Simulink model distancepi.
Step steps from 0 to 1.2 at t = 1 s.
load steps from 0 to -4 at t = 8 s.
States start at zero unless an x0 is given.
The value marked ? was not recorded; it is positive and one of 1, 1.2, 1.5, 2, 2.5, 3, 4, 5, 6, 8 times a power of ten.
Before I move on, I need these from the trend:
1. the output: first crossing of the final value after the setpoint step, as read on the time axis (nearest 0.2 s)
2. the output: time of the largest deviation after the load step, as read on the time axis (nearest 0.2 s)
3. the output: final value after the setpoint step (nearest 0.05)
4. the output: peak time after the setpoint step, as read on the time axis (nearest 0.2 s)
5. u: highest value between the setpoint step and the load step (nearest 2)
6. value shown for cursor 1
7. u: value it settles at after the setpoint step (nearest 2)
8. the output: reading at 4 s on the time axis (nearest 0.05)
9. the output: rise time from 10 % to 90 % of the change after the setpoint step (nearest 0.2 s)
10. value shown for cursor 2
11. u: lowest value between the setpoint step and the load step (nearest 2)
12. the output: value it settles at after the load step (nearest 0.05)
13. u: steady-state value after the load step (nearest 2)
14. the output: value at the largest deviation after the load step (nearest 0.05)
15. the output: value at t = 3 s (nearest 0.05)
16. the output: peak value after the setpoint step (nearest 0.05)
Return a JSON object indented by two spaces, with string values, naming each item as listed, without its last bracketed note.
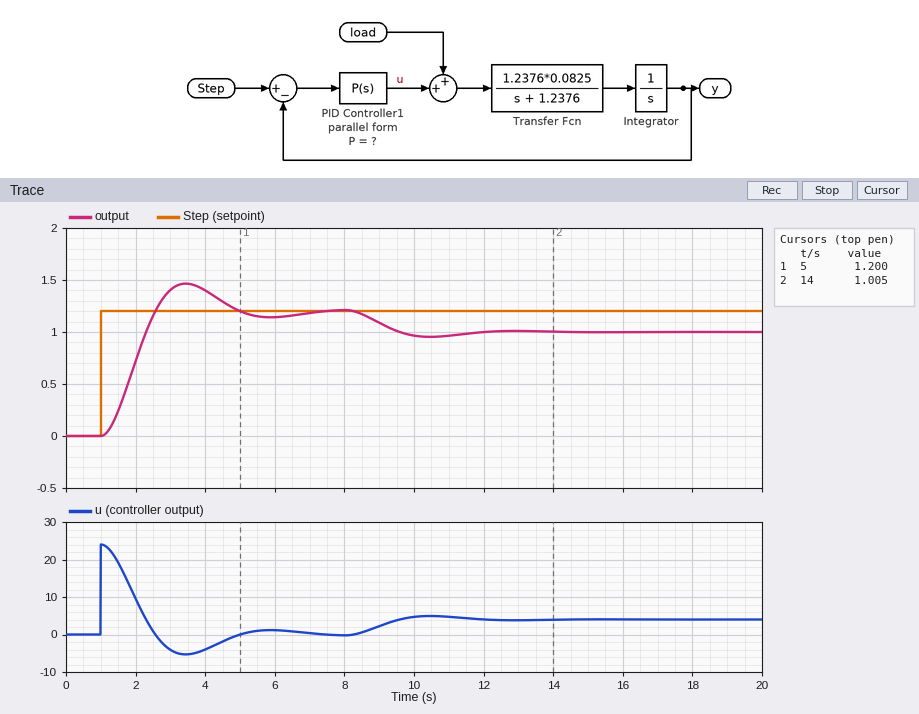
{
  "the output: first crossing of the final value after the setpoint step, as read on the time axis": "2.6 s",
  "the output: time of the largest deviation after the load step, as read on the time axis": "10.4 s",
  "the output: final value after the setpoint step": "1.20",
  "the output: peak time after the setpoint step, as read on the time axis": "3.4 s",
  "u: highest value between the setpoint step and the load step": "24",
  "value shown for cursor 1": "1.200",
  "u: value it settles at after the setpoint step": "0",
  "the output: reading at 4 s on the time axis": "1.40",
  "the output: rise time from 10 % to 90 % of the change after the setpoint step": "1.0 s",
  "value shown for cursor 2": "1.005",
  "u: lowest value between the setpoint step and the load step": "-6",
  "the output: value it settles at after the load step": "1.00",
  "u: steady-state value after the load step": "4",
  "the output: value at the largest deviation after the load step": "0.95",
  "the output: value at t = 3 s": "1.40",
  "the output: peak value after the setpoint step": "1.45"
}
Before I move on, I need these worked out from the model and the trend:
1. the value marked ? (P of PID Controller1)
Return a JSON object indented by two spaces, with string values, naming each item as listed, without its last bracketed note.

{
  "the value marked ?": "20"
}
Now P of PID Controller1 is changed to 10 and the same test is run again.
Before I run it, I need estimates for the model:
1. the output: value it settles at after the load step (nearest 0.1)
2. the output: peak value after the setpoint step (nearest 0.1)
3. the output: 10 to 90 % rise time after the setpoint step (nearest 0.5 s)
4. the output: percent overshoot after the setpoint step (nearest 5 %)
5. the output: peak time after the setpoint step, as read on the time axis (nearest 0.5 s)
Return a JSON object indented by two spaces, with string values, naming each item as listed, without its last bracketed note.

{
  "the output: value it settles at after the load step": "0.8",
  "the output: peak value after the setpoint step": "1.3",
  "the output: 10 to 90 % rise time after the setpoint step": "2.0 s",
  "the output: percent overshoot after the setpoint step": "10 %",
  "the output: peak time after the setpoint step, as read on the time axis": "5.0 s"
}
